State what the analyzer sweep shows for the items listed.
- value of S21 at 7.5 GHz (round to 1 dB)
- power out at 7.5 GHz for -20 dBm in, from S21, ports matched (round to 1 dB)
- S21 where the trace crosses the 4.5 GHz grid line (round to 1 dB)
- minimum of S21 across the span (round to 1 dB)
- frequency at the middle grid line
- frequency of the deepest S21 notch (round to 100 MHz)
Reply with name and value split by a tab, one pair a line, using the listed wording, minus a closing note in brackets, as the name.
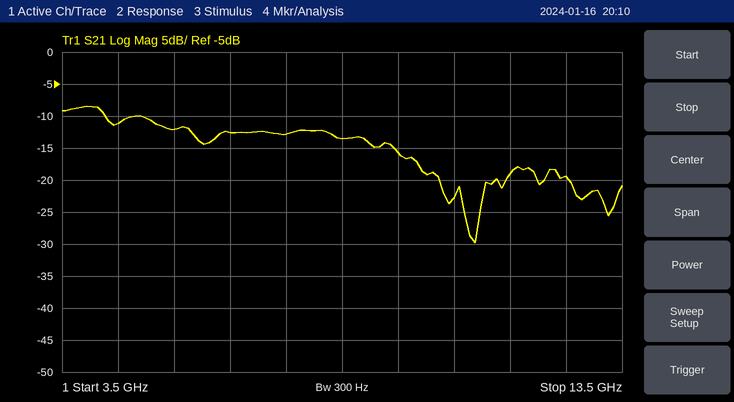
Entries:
value of S21 at 7.5 GHz	-13 dB
power out at 7.5 GHz for -20 dBm in, from S21, ports matched	-33 dBm
S21 where the trace crosses the 4.5 GHz grid line	-11 dB
minimum of S21 across the span	-30 dB
frequency at the middle grid line	8.5 GHz
frequency of the deepest S21 notch	10.9 GHz
